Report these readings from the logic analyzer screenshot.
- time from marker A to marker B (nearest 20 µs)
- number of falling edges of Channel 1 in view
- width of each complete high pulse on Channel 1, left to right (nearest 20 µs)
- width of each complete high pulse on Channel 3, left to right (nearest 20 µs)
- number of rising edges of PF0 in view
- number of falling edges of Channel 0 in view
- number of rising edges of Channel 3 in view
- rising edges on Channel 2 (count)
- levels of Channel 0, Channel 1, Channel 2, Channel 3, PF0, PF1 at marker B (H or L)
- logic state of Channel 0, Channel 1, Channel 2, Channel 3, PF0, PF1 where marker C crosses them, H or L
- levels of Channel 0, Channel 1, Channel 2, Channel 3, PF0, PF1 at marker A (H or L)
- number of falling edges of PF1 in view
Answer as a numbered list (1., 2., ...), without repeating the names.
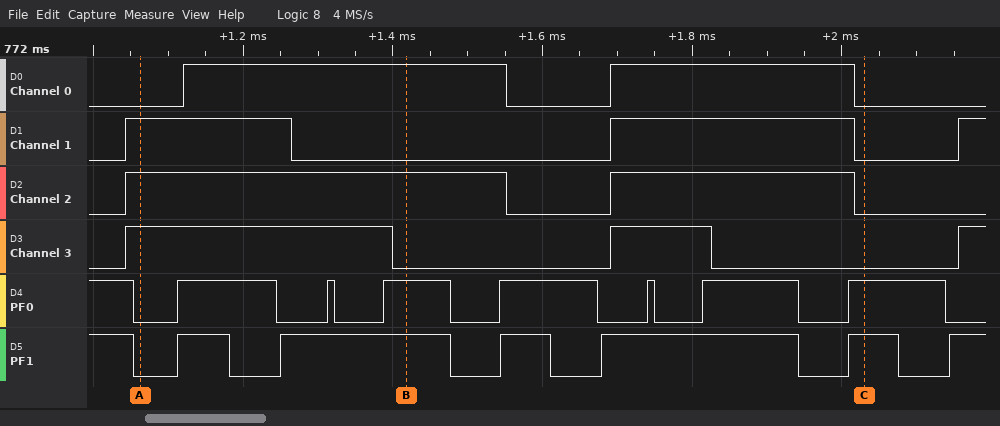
1. 360 µs
2. 2
3. 220 µs, 320 µs
4. 360 µs, 140 µs
5. 7
6. 2
7. 3
8. 2
9. Channel 0=H, Channel 1=L, Channel 2=H, Channel 3=L, PF0=H, PF1=H
10. Channel 0=L, Channel 1=L, Channel 2=L, Channel 3=L, PF0=H, PF1=H
11. Channel 0=L, Channel 1=H, Channel 2=H, Channel 3=H, PF0=L, PF1=L
12. 6
